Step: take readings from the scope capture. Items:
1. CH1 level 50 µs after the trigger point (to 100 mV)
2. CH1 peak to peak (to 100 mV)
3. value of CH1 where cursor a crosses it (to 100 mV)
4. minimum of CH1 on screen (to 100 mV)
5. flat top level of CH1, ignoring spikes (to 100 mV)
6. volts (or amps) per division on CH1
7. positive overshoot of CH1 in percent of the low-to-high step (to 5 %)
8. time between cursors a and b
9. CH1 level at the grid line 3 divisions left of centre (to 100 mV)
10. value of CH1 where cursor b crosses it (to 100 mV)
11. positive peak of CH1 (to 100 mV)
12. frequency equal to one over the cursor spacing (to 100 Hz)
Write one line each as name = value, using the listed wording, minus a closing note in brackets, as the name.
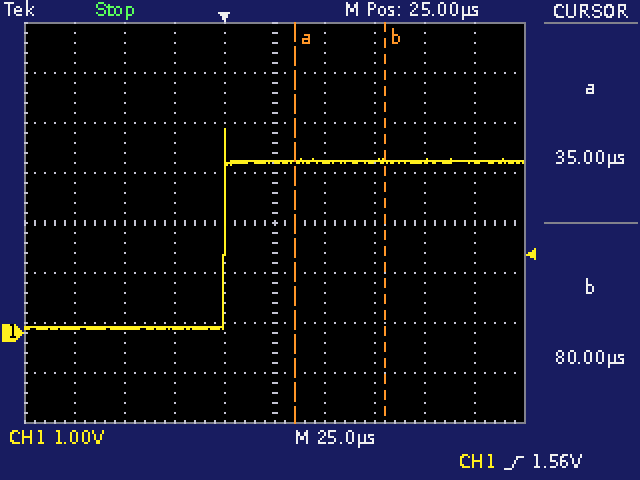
CH1 level 50 µs after the trigger point = 3.4 V
CH1 peak to peak = 4.0 V
value of CH1 where cursor a crosses it = 3.4 V
minimum of CH1 on screen = 100 mV
flat top level of CH1, ignoring spikes = 3.4 V
volts (or amps) per division on CH1 = 1 V
positive overshoot of CH1 in percent of the low-to-high step = 20 %
time between cursors a and b = 45.0 µs
CH1 level at the grid line 3 divisions left of centre = 100 mV
value of CH1 where cursor b crosses it = 3.4 V
positive peak of CH1 = 4.1 V
frequency equal to one over the cursor spacing = 22.2 kHz
